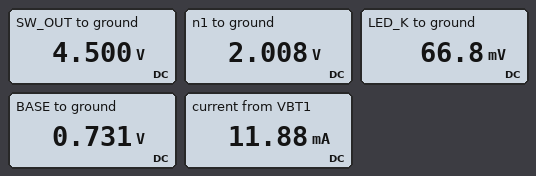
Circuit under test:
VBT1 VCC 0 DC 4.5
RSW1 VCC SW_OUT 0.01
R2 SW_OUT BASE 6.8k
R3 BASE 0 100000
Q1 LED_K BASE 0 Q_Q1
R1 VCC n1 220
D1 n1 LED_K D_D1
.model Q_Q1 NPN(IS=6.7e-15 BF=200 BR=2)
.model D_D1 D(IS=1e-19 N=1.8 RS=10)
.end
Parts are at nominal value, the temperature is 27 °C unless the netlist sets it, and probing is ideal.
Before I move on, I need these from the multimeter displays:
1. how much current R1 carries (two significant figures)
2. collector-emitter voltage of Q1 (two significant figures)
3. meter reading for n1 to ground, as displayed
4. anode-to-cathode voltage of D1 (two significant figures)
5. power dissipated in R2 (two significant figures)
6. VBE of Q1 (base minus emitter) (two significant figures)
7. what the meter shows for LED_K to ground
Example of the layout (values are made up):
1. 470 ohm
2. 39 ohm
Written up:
1. 11 mA
2. 67 mV
3. 2.008 V
4. 1.9 V
5. 2.1 mW
6. 730 mV
7. 66.8 mV
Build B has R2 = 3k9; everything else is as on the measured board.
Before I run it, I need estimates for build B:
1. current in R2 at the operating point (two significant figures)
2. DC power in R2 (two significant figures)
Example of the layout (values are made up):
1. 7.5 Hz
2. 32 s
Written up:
1. 970 µA
2. 3.6 mW
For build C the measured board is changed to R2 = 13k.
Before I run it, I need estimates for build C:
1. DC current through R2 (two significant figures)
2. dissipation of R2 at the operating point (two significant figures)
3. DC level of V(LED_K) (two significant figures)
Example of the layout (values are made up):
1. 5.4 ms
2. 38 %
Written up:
1. 290 µA
2. 1.1 mW
3. 85 mV
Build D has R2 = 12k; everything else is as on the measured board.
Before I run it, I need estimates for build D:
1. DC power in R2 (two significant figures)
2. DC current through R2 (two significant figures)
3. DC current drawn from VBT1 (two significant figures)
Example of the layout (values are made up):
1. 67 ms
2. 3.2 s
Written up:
1. 1.2 mW
2. 310 µA
3. 12 mA
